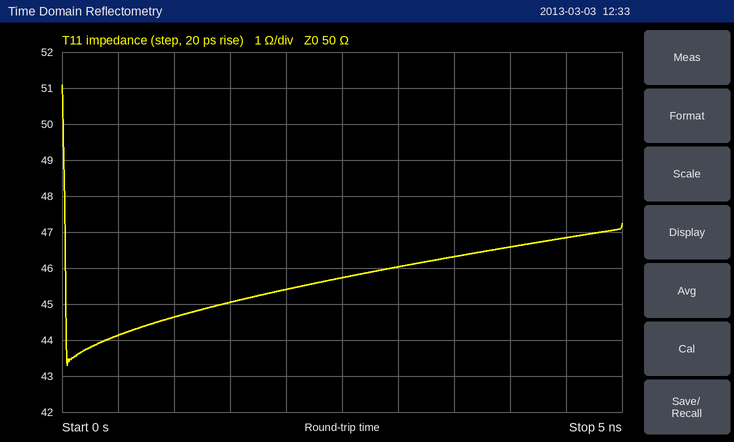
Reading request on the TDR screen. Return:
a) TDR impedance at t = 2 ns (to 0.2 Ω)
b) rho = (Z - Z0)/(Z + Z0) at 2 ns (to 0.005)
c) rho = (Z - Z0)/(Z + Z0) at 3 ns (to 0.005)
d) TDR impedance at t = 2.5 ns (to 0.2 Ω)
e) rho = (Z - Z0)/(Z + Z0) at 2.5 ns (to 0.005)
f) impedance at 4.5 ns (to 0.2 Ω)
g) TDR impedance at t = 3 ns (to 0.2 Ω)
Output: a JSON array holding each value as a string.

["45.4 Ω", "-0.050", "-0.040", "45.8 Ω", "-0.045", "46.8 Ω", "46.0 Ω"]
